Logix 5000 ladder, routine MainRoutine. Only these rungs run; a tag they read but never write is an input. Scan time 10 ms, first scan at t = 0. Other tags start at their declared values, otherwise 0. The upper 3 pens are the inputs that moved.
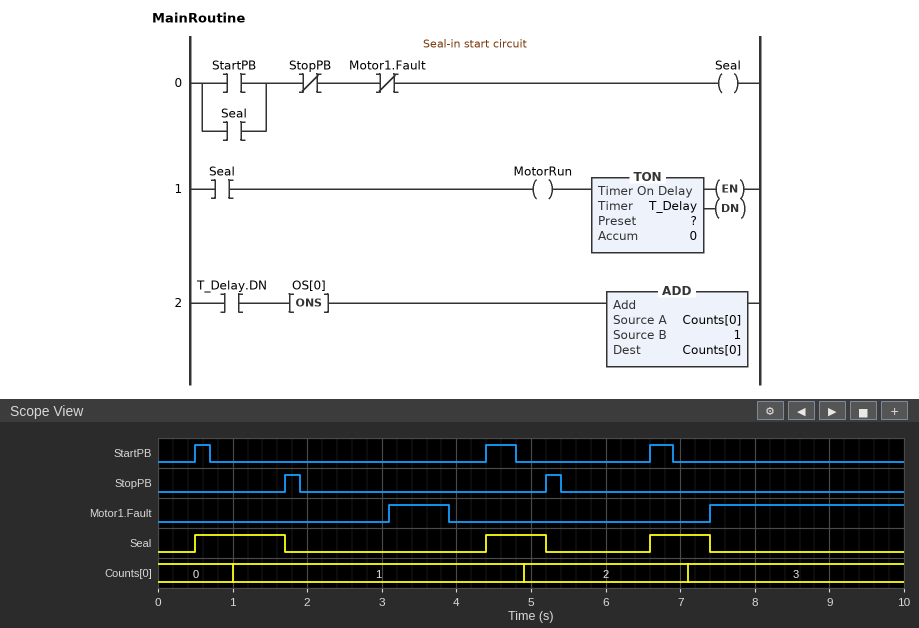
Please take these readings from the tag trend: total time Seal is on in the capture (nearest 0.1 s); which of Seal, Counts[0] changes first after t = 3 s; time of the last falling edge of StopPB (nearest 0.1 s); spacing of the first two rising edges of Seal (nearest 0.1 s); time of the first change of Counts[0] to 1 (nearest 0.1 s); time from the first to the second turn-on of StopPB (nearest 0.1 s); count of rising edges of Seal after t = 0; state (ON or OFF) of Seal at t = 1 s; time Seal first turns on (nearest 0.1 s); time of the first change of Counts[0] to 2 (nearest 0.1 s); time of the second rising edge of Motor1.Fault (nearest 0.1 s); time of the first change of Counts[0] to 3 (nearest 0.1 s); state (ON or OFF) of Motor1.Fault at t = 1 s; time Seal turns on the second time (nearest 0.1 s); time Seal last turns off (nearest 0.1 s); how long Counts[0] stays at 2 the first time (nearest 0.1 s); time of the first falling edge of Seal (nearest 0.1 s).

2.8 s
Seal
5.4 s
3.9 s
1.0 s
3.5 s
3
ON
0.5 s
4.9 s
7.4 s
7.1 s
OFF
4.4 s
7.4 s
2.2 s
1.7 s
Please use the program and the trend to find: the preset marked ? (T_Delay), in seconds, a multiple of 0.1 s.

0.5 s
